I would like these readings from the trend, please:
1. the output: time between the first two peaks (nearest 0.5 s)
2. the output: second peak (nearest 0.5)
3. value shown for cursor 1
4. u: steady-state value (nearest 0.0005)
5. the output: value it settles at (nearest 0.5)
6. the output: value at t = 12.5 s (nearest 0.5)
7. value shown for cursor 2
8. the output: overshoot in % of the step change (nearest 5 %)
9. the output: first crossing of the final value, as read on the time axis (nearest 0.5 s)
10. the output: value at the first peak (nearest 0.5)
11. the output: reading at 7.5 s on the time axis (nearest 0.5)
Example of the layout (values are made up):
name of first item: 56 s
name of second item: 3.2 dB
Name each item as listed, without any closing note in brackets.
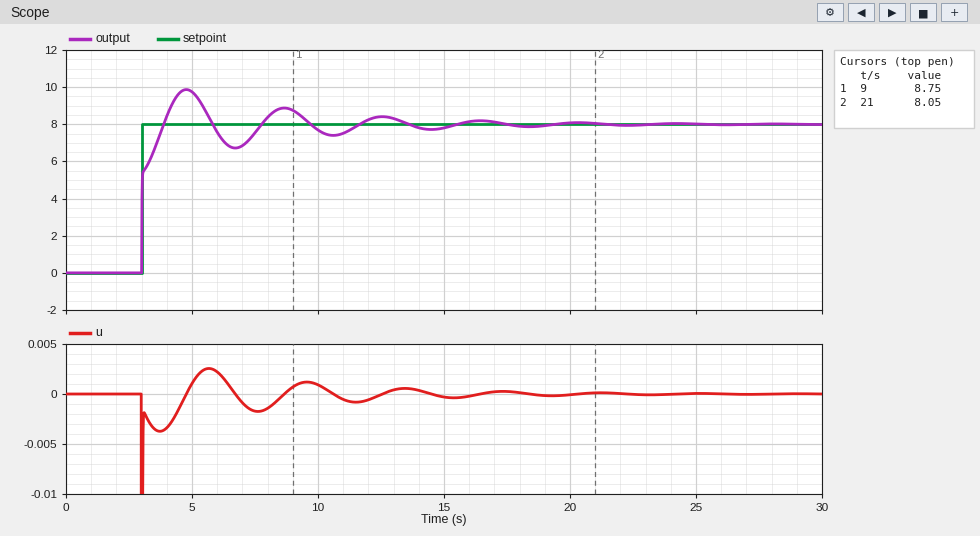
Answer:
the output: time between the first two peaks: 4.0 s
the output: second peak: 9.0
value shown for cursor 1: 8.75
u: steady-state value: 0.0000
the output: value it settles at: 8.0
the output: value at t = 12.5 s: 8.5
value shown for cursor 2: 8.05
the output: overshoot in % of the step change: 25 %
the output: first crossing of the final value, as read on the time axis: 4.0 s
the output: value at the first peak: 10.0
the output: reading at 7.5 s on the time axis: 7.5
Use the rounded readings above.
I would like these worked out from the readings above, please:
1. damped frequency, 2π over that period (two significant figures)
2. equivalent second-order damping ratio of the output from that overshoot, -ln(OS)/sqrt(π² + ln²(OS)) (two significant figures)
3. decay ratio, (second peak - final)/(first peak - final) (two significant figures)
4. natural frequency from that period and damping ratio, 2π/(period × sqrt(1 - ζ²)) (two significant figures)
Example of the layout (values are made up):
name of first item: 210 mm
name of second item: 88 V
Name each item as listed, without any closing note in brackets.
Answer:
damped frequency, 2π over that period: 1.6 rad/s
equivalent second-order damping ratio of the output from that overshoot, -ln(OS)/sqrt(π² + ln²(OS)): 0.40
decay ratio, (second peak - final)/(first peak - final): 0.50
natural frequency from that period and damping ratio, 2π/(period × sqrt(1 - ζ²)): 1.7 rad/s
